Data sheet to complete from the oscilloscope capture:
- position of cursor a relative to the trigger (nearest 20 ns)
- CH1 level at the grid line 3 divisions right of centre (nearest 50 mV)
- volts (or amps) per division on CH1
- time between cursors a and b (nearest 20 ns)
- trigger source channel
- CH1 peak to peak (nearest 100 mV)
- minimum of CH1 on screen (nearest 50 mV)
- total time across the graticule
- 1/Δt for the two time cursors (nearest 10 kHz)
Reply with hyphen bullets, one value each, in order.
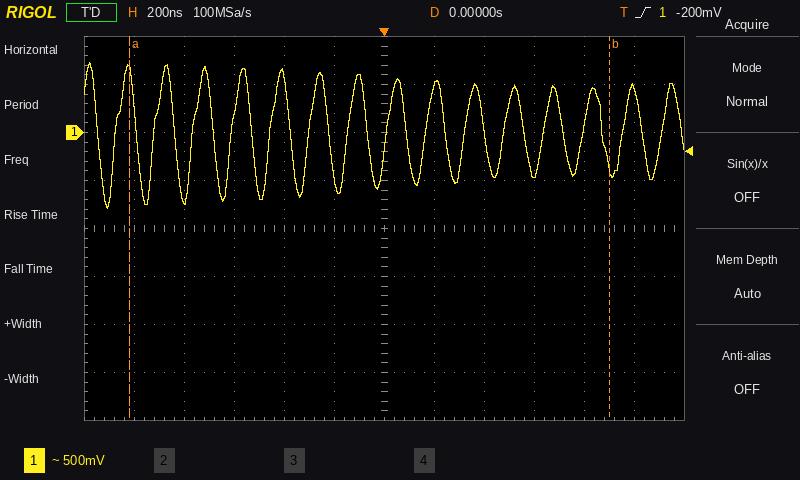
- -1.02 µs
- -450 mV
- 500 mV
- 1.92 µs
- CH1
- 1.50 V
- -800 mV
- 2.4 µs
- 520 kHz
